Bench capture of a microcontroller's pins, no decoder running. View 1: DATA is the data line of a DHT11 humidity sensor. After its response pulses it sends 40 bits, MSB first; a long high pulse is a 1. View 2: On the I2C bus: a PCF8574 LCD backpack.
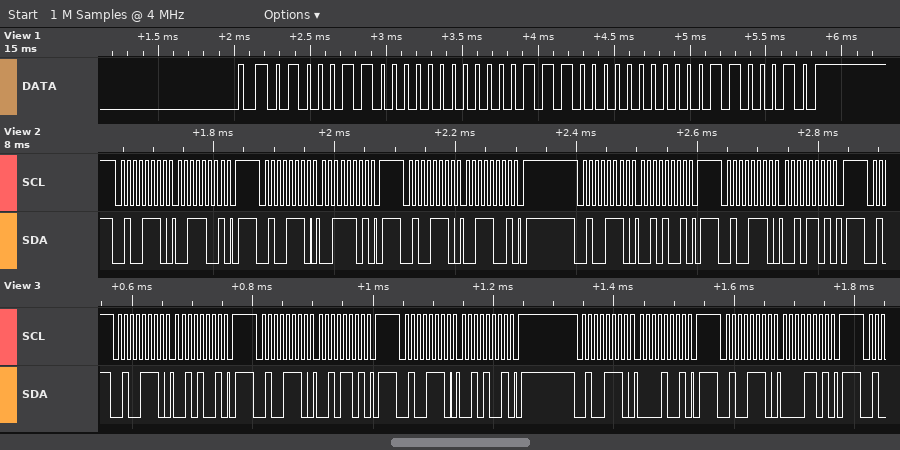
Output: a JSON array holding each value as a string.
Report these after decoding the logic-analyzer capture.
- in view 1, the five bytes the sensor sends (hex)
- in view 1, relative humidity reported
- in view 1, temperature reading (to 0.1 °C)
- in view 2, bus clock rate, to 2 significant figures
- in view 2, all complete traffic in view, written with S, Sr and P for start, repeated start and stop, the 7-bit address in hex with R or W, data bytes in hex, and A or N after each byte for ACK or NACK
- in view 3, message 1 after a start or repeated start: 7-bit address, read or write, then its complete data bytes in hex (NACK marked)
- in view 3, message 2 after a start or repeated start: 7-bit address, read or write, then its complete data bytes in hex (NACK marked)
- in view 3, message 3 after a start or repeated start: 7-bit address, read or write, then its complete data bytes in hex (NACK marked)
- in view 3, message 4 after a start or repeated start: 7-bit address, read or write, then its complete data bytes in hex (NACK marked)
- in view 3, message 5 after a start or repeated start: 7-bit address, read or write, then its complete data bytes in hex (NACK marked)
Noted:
["46 00 1C 00 62", "70 %", "28.0 °C", "100 kHz", "S 27W A 39 A P S 27W A 3D A P S 27W A 39 A P S 27W A 29 A P S 27W A 2D A P", "0x27 write: 29", "0x27 write: 2D", "0x27 write: 29", "0x27 write: 09", "0x27 write: 0D"]
